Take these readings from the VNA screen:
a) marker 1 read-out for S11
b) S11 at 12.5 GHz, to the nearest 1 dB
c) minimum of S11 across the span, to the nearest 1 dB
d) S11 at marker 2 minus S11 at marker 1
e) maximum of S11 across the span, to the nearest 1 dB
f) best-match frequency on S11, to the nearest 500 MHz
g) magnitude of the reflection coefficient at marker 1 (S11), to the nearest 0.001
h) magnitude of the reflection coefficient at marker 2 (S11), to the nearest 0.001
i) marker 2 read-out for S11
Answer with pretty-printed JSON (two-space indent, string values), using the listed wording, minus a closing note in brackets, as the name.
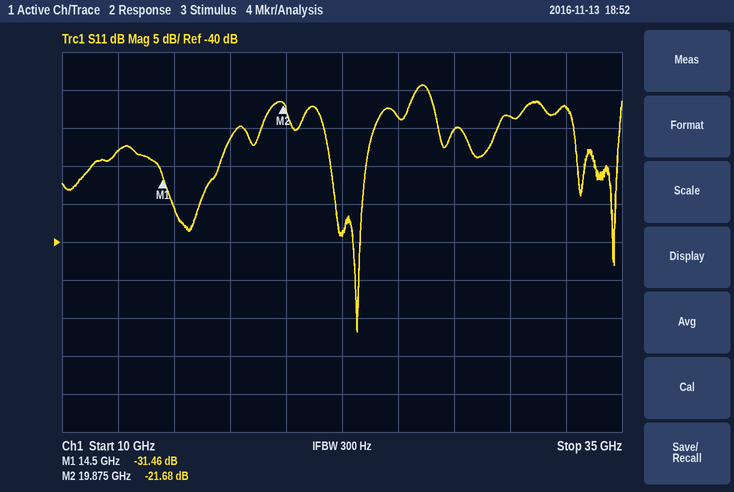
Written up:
{
  "marker 1 read-out for S11": "-31.46 dB",
  "S11 at 12.5 GHz, to the nearest 1 dB": "-28 dB",
  "minimum of S11 across the span, to the nearest 1 dB": "-52 dB",
  "S11 at marker 2 minus S11 at marker 1": "9.78 dB",
  "maximum of S11 across the span, to the nearest 1 dB": "-19 dB",
  "best-match frequency on S11, to the nearest 500 MHz": "23.0 GHz",
  "magnitude of the reflection coefficient at marker 1 (S11), to the nearest 0.001": "0.027",
  "magnitude of the reflection coefficient at marker 2 (S11), to the nearest 0.001": "0.082",
  "marker 2 read-out for S11": "-21.68 dB"
}
